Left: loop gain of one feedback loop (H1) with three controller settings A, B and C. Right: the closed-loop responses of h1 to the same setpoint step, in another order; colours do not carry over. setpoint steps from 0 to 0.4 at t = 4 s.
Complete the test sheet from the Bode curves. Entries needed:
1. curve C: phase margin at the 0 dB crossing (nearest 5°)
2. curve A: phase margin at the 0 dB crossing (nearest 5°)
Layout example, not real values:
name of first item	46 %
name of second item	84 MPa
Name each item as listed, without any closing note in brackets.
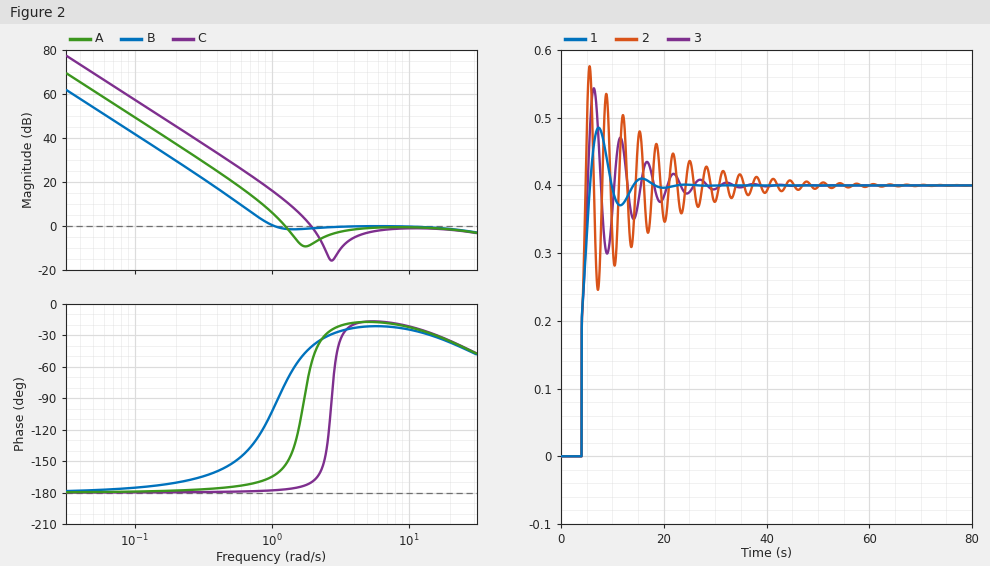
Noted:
curve C: phase margin at the 0 dB crossing	10°
curve A: phase margin at the 0 dB crossing	25°
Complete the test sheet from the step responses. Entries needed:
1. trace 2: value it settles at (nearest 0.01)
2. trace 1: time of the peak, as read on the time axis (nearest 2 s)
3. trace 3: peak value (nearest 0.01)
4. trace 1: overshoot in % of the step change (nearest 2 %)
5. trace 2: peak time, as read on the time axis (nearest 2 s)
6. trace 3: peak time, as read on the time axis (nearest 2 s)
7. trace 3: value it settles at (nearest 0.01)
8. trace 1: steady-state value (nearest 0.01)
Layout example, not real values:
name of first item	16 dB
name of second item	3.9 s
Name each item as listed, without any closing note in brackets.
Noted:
trace 2: value it settles at	0.40
trace 1: time of the peak, as read on the time axis	8 s
trace 3: peak value	0.54
trace 1: overshoot in % of the step change	22 %
trace 2: peak time, as read on the time axis	6 s
trace 3: peak time, as read on the time axis	6 s
trace 3: value it settles at	0.40
trace 1: steady-state value	0.40
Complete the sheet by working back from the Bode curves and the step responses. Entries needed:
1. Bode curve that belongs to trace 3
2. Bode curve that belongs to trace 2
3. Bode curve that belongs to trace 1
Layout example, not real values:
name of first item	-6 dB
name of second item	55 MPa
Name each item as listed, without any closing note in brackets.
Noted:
Bode curve that belongs to trace 3	A
Bode curve that belongs to trace 2	C
Bode curve that belongs to trace 1	B
